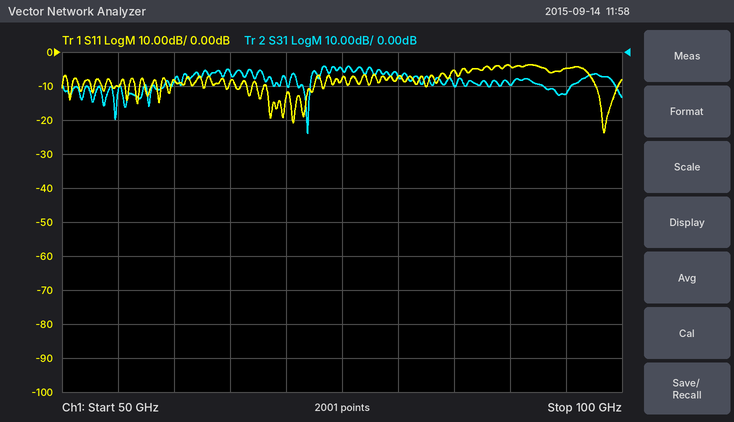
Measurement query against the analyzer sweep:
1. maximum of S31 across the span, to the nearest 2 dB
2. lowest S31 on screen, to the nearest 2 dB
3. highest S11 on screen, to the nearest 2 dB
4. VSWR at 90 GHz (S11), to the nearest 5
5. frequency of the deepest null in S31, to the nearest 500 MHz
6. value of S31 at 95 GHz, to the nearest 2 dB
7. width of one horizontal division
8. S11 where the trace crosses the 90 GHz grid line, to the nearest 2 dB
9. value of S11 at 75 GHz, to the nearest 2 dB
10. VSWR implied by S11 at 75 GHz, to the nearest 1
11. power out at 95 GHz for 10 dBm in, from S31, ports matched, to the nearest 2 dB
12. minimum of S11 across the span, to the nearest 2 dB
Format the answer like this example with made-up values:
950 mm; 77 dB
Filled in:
-4 dB; -24 dB; -4 dB; 5; 72.0 GHz; -12 dB; 5 GHz; -4 dB; -8 dB; 2; -2 dBm; -24 dB
